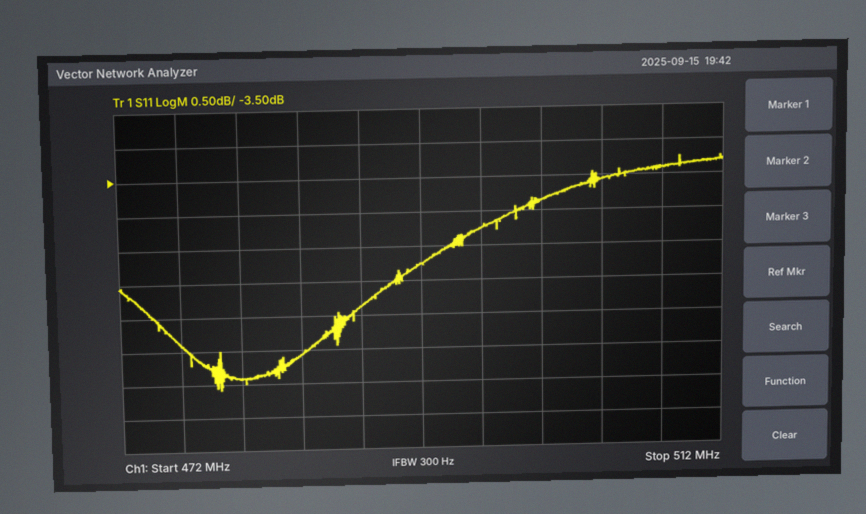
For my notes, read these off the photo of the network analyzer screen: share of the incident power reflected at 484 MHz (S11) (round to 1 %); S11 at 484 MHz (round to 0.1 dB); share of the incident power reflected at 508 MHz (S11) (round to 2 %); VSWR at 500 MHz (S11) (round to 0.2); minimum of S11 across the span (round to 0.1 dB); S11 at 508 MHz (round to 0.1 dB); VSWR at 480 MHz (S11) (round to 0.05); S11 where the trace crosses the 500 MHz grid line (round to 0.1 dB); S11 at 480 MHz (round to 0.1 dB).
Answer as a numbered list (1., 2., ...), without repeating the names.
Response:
1. 25 %
2. -6.1 dB
3. 46 %
4. 4.6
5. -6.6 dB
6. -3.4 dB
7. 2.85
8. -3.9 dB
9. -6.4 dB
